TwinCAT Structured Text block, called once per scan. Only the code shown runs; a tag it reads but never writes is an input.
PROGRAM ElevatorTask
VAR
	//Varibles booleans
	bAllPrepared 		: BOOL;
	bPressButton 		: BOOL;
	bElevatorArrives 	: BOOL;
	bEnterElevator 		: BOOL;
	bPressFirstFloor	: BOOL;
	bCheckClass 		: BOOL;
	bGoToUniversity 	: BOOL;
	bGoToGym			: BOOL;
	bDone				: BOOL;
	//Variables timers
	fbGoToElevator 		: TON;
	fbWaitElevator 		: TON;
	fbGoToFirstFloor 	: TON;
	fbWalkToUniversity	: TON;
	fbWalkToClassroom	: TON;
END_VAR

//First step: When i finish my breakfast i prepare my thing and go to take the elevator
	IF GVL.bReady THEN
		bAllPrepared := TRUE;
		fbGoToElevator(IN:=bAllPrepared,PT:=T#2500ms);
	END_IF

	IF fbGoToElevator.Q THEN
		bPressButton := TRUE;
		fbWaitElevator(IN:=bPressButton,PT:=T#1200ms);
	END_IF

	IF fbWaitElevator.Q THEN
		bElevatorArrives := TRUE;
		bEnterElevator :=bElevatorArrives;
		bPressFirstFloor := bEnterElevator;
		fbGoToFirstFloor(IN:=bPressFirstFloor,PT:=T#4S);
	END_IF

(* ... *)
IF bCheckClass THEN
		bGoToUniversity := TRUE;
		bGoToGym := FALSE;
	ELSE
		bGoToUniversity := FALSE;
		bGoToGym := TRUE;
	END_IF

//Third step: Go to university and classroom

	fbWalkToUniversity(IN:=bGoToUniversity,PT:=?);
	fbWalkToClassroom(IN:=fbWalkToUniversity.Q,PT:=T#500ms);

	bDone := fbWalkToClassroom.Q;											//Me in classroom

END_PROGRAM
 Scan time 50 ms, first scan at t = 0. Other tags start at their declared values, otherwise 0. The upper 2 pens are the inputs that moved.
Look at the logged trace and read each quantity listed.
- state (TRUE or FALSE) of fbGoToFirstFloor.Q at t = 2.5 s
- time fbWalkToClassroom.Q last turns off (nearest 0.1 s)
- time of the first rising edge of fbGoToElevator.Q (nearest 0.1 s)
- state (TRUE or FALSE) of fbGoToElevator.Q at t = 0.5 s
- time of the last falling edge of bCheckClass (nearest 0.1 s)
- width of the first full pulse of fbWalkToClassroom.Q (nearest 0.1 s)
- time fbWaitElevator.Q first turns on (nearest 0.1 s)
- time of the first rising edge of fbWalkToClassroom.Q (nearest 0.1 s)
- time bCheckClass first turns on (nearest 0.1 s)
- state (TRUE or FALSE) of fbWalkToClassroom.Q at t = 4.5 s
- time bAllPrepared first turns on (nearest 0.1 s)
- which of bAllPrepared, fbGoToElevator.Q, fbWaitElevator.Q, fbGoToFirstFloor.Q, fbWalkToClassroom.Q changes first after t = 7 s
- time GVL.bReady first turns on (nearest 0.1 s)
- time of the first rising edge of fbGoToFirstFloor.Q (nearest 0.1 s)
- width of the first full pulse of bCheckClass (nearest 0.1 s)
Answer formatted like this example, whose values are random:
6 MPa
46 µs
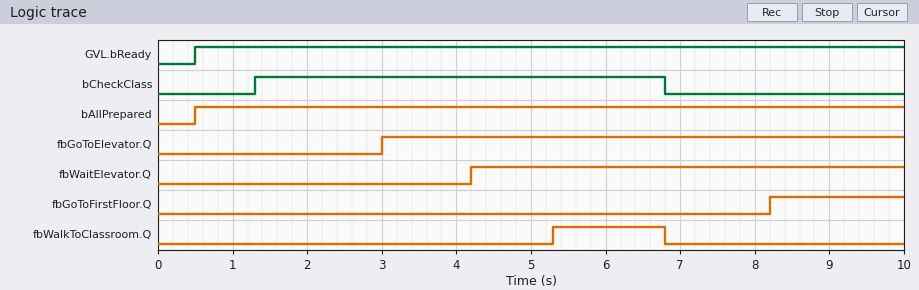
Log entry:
FALSE
6.8 s
3.0 s
FALSE
6.8 s
1.5 s
4.2 s
5.3 s
1.3 s
FALSE
0.5 s
fbGoToFirstFloor.Q
0.5 s
8.2 s
5.5 s
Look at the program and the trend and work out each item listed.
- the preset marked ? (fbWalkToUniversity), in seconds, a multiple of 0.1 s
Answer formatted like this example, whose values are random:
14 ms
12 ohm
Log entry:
3.5 s
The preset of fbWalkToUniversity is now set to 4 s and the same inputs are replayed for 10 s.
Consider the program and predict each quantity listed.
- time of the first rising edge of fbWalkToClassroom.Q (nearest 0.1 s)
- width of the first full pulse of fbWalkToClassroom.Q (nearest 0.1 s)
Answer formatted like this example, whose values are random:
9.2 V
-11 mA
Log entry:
5.8 s
1.0 s
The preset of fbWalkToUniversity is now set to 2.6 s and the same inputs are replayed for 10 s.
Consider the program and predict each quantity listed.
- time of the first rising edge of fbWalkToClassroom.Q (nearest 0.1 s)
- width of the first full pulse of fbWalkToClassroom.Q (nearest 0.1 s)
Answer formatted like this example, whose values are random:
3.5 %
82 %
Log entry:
4.4 s
2.4 s
